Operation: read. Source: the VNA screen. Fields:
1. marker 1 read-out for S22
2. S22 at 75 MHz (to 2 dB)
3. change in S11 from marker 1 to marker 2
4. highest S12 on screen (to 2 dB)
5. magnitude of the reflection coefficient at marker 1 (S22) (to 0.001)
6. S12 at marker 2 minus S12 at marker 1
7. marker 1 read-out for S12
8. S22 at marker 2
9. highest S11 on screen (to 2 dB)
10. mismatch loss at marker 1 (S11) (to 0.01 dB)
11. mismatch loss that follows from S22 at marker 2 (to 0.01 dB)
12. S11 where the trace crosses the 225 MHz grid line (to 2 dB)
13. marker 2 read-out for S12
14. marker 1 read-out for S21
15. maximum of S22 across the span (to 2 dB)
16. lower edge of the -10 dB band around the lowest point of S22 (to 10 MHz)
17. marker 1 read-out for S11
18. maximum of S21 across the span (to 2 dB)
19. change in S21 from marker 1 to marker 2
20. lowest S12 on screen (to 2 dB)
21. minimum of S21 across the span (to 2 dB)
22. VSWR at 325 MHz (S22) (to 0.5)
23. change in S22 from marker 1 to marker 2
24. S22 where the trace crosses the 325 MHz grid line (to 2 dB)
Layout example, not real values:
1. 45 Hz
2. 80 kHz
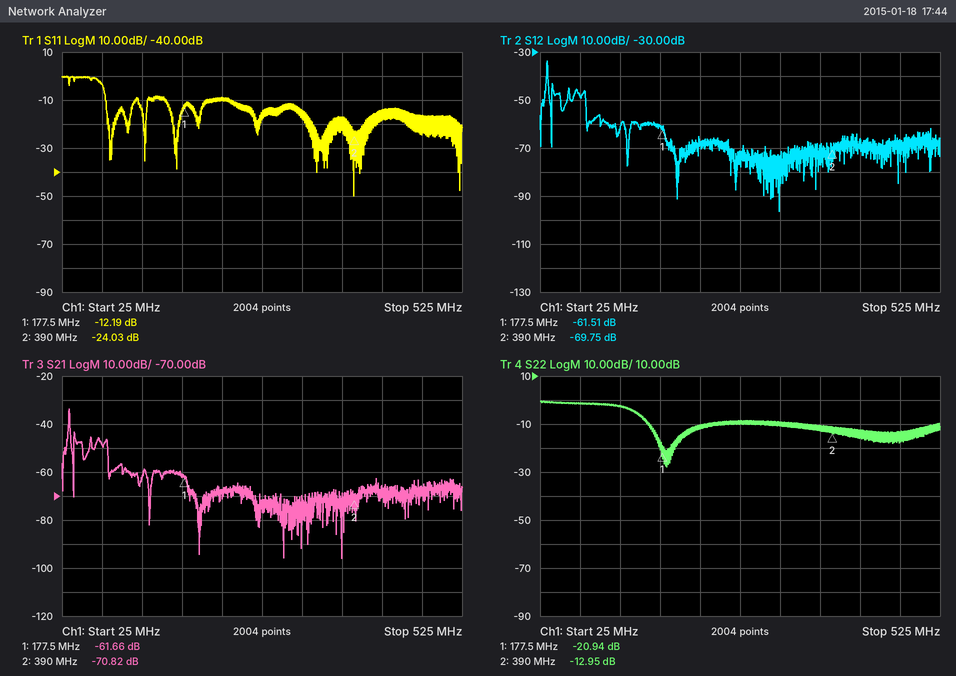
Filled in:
1. -20.94 dB
2. -2 dB
3. -11.84 dB
4. -34 dB
5. 0.090
6. -8.24 dB
7. -61.51 dB
8. -12.95 dB
9. 0 dB
10. 0.27 dB
11. 0.23 dB
12. -10 dB
13. -69.75 dB
14. -61.66 dB
15. 0 dB
16. 160 MHz
17. -12.19 dB
18. -34 dB
19. -9.16 dB
20. -96 dB
21. -96 dB
22. 2.0
23. 7.99 dB
24. -10 dB
